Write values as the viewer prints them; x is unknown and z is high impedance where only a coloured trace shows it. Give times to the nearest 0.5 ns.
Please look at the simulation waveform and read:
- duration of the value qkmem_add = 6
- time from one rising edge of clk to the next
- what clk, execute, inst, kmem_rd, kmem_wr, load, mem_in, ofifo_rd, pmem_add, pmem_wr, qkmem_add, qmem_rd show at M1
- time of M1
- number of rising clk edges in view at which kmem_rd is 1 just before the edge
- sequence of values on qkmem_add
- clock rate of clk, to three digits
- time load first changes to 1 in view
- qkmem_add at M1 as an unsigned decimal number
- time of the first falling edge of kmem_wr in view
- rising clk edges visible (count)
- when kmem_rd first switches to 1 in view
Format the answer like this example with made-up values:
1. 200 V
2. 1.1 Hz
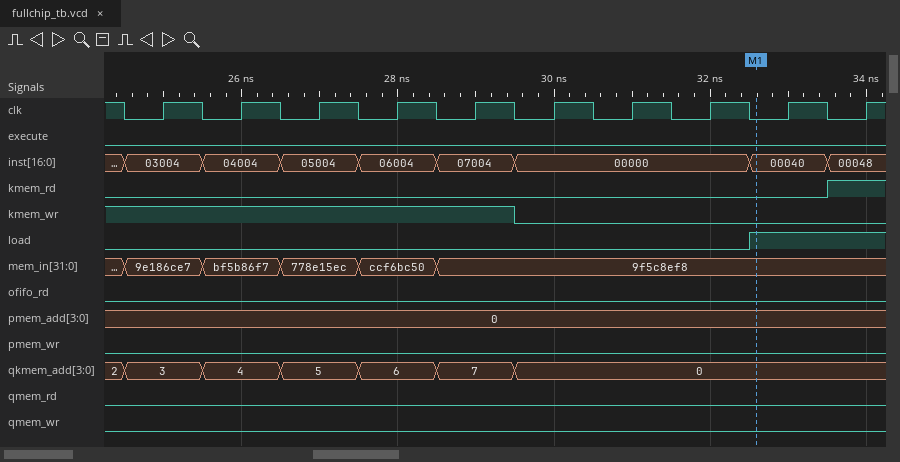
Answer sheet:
1. 1 ns
2. 1 ns
3. clk=0, execute=0, inst=00040, kmem_rd=0, kmem_wr=0, load=1, mem_in=9f5c8ef8, ofifo_rd=0, pmem_add=0, pmem_wr=0, qkmem_add=0, qmem_rd=0
4. 32.5 ns
5. 1
6. 2, 3, 4, 5, 6, 7, 0
7. 1.00 GHz
8. 32.5 ns
9. 0
10. 29.5 ns
11. 10
12. 33.5 ns
